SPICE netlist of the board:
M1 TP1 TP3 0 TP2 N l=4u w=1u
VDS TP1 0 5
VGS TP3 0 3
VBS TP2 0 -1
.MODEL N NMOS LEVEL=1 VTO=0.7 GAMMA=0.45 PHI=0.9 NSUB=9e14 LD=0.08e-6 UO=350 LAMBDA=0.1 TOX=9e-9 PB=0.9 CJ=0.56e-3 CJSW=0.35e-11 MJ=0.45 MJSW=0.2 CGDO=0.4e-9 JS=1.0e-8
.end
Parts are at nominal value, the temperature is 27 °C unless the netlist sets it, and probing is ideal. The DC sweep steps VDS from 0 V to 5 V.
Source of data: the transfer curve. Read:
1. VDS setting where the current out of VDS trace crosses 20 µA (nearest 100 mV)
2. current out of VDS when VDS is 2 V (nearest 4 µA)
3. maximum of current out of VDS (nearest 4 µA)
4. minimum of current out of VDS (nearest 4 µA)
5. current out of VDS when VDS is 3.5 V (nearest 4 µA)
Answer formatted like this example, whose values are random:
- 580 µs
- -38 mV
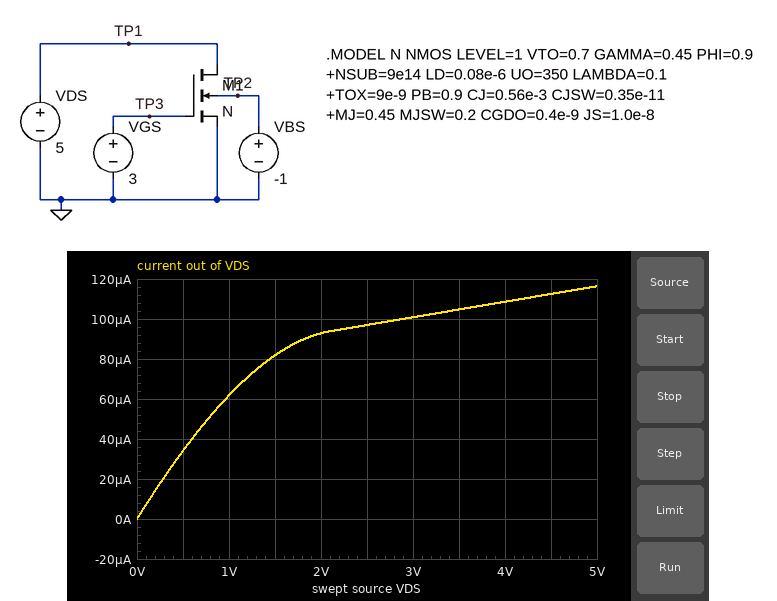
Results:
- 300 mV
- 92 µA
- 116 µA
- 0 A
- 104 µA
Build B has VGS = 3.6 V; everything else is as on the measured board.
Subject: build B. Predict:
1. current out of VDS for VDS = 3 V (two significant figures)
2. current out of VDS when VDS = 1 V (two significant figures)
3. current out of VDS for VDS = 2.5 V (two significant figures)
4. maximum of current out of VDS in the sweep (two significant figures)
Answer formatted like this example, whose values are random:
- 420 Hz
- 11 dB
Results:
- 170 µA
- 85 µA
- 160 µA
- 190 µA
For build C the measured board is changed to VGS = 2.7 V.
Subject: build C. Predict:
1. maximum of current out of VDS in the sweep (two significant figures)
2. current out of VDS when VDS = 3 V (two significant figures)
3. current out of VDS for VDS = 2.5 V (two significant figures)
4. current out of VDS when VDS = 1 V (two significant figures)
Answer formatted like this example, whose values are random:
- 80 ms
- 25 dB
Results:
- 86 µA
- 74 µA
- 71 µA
- 50 µA
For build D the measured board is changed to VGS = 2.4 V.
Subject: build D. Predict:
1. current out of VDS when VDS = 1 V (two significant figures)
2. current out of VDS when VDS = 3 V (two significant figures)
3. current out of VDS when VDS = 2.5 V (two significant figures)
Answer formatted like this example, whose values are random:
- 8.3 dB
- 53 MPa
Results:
- 39 µA
- 52 µA
- 50 µA
